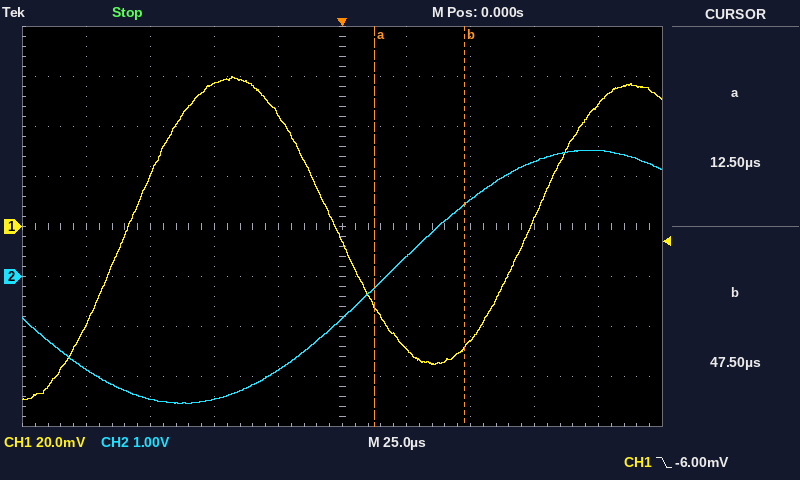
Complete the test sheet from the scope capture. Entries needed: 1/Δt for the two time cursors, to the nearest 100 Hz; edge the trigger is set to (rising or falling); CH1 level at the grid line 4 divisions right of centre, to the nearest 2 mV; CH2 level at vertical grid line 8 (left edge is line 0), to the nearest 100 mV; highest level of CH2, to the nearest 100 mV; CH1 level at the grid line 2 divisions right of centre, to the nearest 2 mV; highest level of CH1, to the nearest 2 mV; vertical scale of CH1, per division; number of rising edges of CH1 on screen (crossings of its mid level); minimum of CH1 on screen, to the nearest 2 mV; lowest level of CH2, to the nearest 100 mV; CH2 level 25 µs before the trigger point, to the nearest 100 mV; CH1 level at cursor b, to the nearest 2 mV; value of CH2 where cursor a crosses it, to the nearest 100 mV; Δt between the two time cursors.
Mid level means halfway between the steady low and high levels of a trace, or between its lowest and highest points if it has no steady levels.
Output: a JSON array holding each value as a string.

["28.6 kHz", "falling", "48 mV", "2.3 V", "2.5 V", "-46 mV", "60 mV", "20 mV", "2", "-70 mV", "-2.5 V", "-1.9 V", "-48 mV", "-200 mV", "35.0 µs"]
